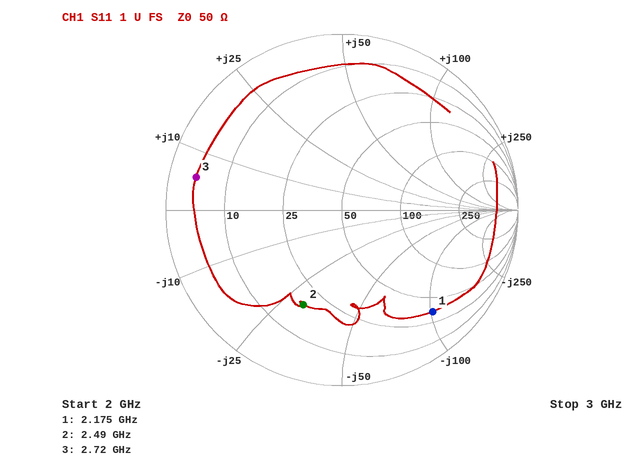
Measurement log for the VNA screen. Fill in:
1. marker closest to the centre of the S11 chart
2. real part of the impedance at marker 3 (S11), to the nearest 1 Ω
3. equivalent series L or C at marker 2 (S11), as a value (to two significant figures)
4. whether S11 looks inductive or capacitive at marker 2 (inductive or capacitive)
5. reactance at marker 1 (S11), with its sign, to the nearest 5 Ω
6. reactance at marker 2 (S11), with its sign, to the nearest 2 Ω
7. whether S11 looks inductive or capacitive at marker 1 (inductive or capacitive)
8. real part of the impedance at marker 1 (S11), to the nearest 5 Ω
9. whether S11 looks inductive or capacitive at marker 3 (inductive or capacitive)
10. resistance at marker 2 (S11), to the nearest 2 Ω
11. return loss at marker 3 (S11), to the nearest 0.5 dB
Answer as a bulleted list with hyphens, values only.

- marker 2
- 4 Ω
- 2.1 pF
- capacitive
- -100 Ω
- -30 Ω
- capacitive
- 35 Ω
- inductive
- 18 Ω
- 1.5 dB
